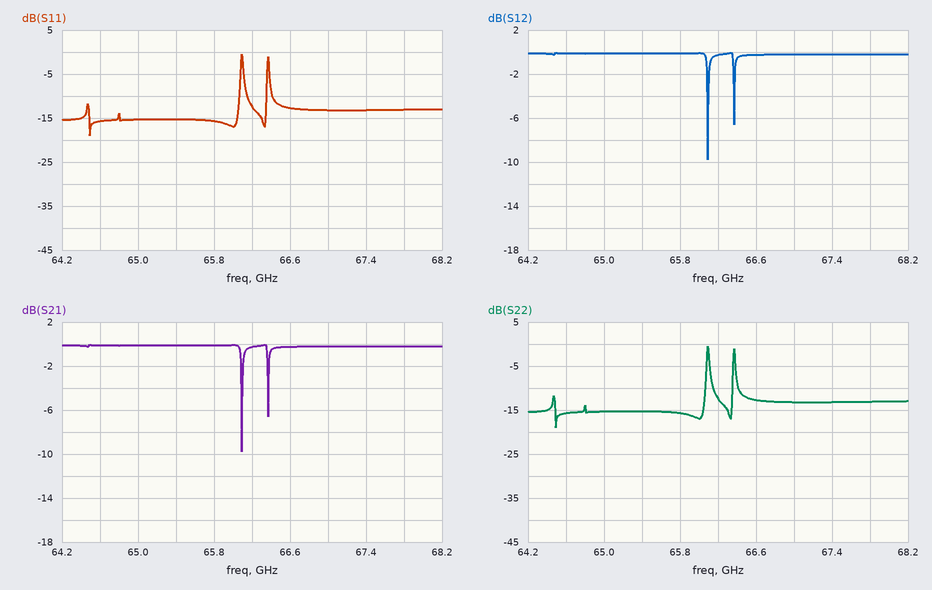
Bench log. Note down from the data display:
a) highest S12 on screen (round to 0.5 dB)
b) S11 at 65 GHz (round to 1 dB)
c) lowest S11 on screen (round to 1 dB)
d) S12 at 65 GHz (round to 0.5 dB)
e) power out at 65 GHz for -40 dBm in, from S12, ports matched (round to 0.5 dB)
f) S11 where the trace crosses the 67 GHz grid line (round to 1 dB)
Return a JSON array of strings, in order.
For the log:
["0.0 dB", "-15 dB", "-19 dB", "0.0 dB", "-40.0 dBm", "-13 dB"]
